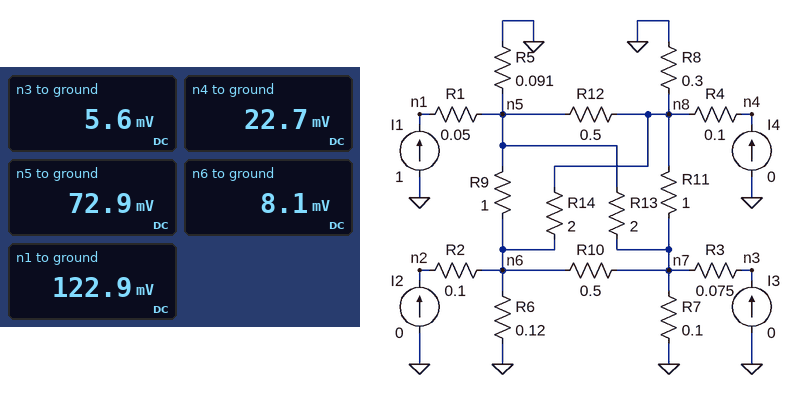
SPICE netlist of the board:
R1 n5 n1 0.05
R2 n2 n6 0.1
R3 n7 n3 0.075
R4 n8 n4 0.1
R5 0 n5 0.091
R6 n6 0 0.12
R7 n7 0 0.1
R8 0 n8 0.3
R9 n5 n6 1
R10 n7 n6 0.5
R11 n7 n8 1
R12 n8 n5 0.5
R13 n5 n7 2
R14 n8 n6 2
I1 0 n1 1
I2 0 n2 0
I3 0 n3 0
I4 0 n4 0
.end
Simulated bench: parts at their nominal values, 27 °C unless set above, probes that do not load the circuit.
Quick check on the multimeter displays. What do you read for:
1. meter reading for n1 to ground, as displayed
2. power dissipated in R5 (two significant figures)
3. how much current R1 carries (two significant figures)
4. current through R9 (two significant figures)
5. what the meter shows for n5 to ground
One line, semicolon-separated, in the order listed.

122.9 mV; 58 mW; 1.0 A; 65 mA; 72.9 mV
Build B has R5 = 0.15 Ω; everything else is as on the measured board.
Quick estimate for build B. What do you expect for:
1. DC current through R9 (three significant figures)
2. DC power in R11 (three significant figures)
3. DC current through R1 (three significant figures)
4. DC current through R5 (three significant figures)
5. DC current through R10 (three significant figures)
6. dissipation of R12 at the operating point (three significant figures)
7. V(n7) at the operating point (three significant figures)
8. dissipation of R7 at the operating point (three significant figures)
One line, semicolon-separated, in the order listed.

94.7 mA; 628 µW; 1.00 A; 710 mA; 7.26 mA; 10.7 mW; 8.15 mV; 664 µW
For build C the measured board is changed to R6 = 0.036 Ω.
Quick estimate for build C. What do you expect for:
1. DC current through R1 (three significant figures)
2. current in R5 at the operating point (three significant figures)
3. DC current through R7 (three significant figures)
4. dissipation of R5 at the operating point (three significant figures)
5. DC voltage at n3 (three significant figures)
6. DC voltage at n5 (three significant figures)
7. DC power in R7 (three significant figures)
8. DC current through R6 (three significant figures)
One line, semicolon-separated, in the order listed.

1.00 A; 796 mA; 47.6 mA; 57.7 mW; 4.76 mV; 72.4 mV; 227 µW; 82.6 mA
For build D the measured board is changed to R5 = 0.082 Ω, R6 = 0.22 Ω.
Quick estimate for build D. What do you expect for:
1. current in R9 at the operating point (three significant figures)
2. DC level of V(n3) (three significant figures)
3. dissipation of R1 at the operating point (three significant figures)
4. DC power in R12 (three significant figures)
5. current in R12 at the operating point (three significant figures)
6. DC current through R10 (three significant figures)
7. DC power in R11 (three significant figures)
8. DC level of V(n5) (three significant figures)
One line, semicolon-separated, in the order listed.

56.2 mA; 5.72 mV; 50.0 mW; 4.23 mW; 91.9 mA; 10.8 mA; 244 µW; 67.3 mV
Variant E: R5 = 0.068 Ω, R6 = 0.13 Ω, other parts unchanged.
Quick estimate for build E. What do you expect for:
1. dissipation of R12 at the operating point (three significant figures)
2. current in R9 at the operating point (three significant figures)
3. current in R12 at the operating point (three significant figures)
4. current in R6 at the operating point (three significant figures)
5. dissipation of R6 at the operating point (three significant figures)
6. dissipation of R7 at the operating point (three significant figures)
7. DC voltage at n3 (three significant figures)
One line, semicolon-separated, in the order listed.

3.11 mW; 50.7 mA; 78.9 mA; 51.7 mA; 348 µW; 198 µW; 4.45 mV
